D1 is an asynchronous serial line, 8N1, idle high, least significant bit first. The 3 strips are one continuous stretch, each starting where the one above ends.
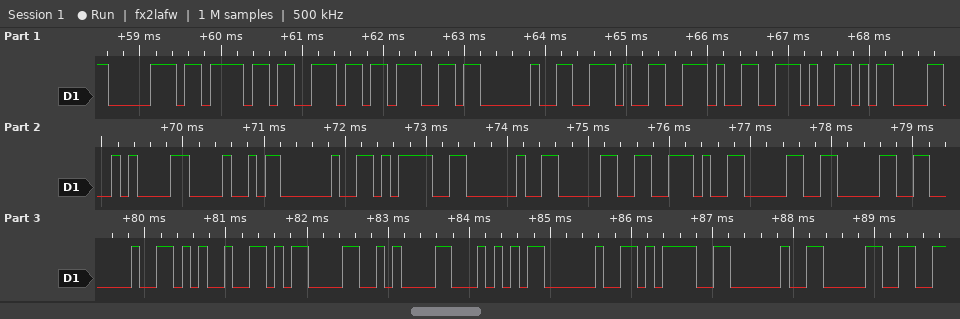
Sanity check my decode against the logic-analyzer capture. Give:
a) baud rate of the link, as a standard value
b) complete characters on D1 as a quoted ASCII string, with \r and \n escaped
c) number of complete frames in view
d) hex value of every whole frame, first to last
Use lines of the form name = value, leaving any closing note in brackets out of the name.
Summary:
baud rate of the link, as a standard value = 9600 baud
complete characters on D1 as a quoted ASCII string, with \r and \n escaped = "pong ...\r\nH = 0.00 %\r\nT = 0"
number of complete frames in view = 27
hex value of every whole frame, first to last = 70 6F 6E 67 20 2E 2E 2E 0D 0A 48 20 3D 20 30 2E 30 30 20 25 0D 0A 54 20 3D 20 30
